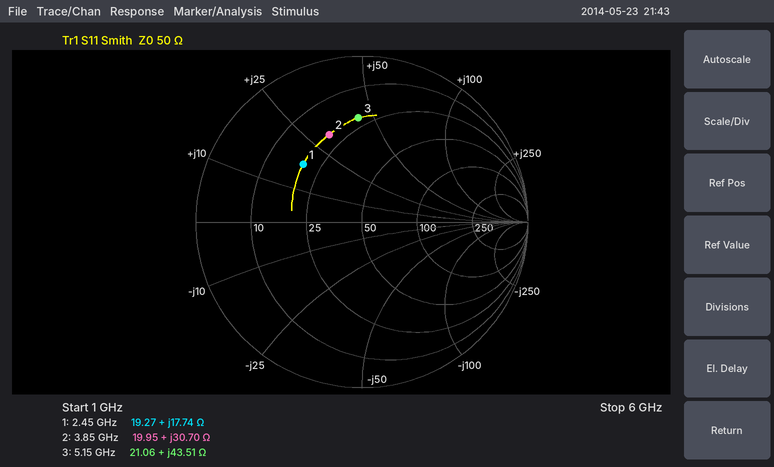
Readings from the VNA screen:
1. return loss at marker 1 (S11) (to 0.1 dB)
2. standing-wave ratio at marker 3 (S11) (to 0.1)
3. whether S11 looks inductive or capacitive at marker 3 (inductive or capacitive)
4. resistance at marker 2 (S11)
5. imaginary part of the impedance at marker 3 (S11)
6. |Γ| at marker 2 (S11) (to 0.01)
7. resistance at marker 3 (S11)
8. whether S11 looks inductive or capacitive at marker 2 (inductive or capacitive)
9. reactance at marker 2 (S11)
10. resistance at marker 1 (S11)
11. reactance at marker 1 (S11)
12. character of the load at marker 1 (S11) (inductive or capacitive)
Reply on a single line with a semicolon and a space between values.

6.1 dB; 4.4; inductive; 19.95 Ω; +43.51 Ω; 0.56; 21.06 Ω; inductive; +30.70 Ω; 19.27 Ω; +17.74 Ω; inductive
